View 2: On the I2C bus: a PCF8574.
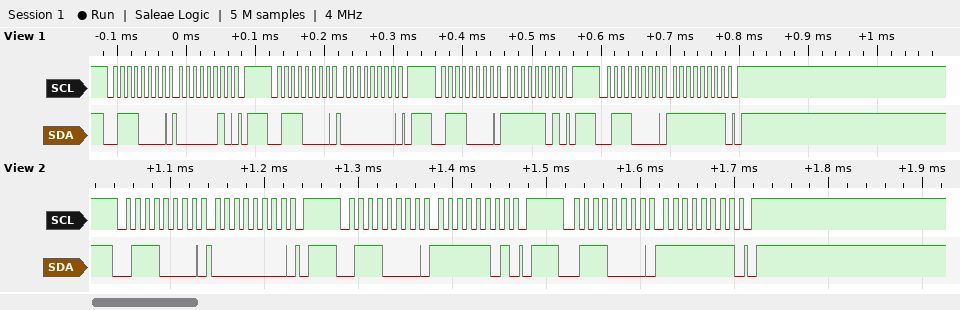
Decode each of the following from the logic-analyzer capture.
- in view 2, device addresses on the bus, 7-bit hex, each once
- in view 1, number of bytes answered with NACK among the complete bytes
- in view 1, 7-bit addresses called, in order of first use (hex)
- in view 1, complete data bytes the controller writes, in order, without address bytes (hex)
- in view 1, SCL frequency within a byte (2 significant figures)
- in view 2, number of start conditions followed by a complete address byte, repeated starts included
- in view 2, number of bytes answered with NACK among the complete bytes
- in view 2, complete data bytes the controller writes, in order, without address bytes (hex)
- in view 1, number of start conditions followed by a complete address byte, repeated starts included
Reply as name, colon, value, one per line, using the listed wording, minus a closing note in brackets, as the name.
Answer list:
in view 2, device addresses on the bus, 7-bit hex, each once: 0x38
in view 1, number of bytes answered with NACK among the complete bytes: 0
in view 1, 7-bit addresses called, in order of first use: 0x38
in view 1, complete data bytes the controller writes, in order, without address bytes: 02 00 FD FF
in view 1, SCL frequency within a byte: 100 kHz
in view 2, number of start conditions followed by a complete address byte, repeated starts included: 3
in view 2, number of bytes answered with NACK among the complete bytes: 0
in view 2, complete data bytes the controller writes, in order, without address bytes: 00 FD FF
in view 1, number of start conditions followed by a complete address byte, repeated starts included: 4
